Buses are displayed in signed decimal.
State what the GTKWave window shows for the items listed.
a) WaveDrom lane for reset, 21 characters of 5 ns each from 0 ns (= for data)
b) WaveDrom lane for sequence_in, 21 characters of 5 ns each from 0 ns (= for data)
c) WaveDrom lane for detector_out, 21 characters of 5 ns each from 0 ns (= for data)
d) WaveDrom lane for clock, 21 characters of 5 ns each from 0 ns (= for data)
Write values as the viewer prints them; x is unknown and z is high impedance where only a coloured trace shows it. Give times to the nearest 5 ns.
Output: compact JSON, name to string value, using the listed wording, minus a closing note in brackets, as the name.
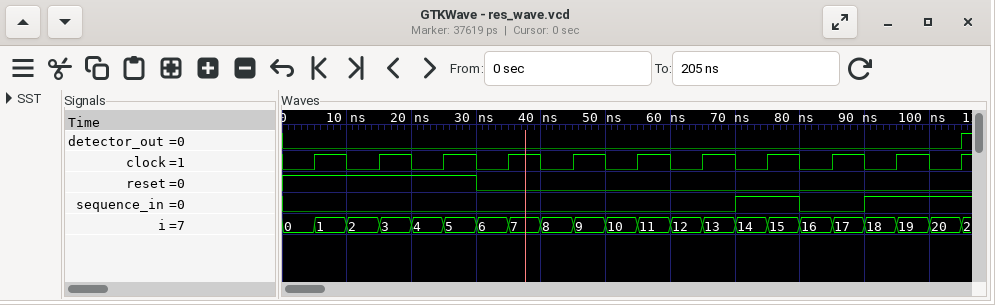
{"WaveDrom lane for reset, 21 characters of 5 ns each from 0 ns": "{name: 'reset', wave: '1.....0..............'}", "WaveDrom lane for sequence_in, 21 characters of 5 ns each from 0 ns": "{name: 'sequence_in', wave: '0.............1.0.1..'}", "WaveDrom lane for detector_out, 21 characters of 5 ns each from 0 ns": "{name: 'detector_out', wave: '0....................'}", "WaveDrom lane for clock, 21 characters of 5 ns each from 0 ns": "{name: 'clock', wave: '010101010101010101010'}"}
